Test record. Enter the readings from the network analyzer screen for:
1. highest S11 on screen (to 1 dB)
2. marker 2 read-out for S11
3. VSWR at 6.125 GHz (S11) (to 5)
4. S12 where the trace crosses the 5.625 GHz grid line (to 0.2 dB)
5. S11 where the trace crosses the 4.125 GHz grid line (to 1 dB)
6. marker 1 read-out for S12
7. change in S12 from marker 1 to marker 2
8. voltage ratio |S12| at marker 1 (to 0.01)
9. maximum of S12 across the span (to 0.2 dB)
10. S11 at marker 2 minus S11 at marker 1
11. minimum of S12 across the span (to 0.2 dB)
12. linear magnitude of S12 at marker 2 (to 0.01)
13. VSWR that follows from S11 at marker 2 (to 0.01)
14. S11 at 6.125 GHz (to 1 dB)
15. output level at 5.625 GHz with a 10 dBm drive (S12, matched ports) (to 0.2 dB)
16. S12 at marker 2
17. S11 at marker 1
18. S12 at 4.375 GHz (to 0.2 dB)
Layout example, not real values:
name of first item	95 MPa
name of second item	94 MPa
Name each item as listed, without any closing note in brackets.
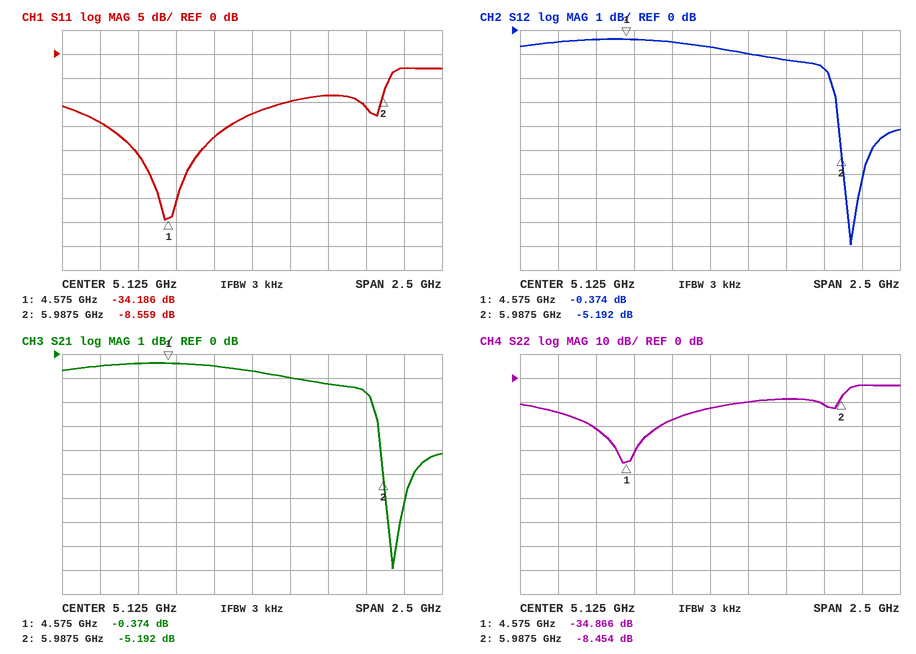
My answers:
highest S11 on screen	-3 dB
marker 2 read-out for S11	-8.559 dB
VSWR at 6.125 GHz (S11)	5
S12 where the trace crosses the 5.625 GHz grid line	-1.2 dB
S11 where the trace crosses the 4.125 GHz grid line	-14 dB
marker 1 read-out for S12	-0.374 dB
change in S12 from marker 1 to marker 2	-4.818 dB
voltage ratio |S12| at marker 1	0.96
maximum of S12 across the span	-0.4 dB
S11 at marker 2 minus S11 at marker 1	25.627 dB
minimum of S12 across the span	-9.0 dB
linear magnitude of S12 at marker 2	0.55
VSWR that follows from S11 at marker 2	2.19
S11 at 6.125 GHz	-3 dB
output level at 5.625 GHz with a 10 dBm drive (S12, matched ports)	8.8 dBm
S12 at marker 2	-5.192 dB
S11 at marker 1	-34.186 dB
S12 at 4.375 GHz	-0.4 dB
